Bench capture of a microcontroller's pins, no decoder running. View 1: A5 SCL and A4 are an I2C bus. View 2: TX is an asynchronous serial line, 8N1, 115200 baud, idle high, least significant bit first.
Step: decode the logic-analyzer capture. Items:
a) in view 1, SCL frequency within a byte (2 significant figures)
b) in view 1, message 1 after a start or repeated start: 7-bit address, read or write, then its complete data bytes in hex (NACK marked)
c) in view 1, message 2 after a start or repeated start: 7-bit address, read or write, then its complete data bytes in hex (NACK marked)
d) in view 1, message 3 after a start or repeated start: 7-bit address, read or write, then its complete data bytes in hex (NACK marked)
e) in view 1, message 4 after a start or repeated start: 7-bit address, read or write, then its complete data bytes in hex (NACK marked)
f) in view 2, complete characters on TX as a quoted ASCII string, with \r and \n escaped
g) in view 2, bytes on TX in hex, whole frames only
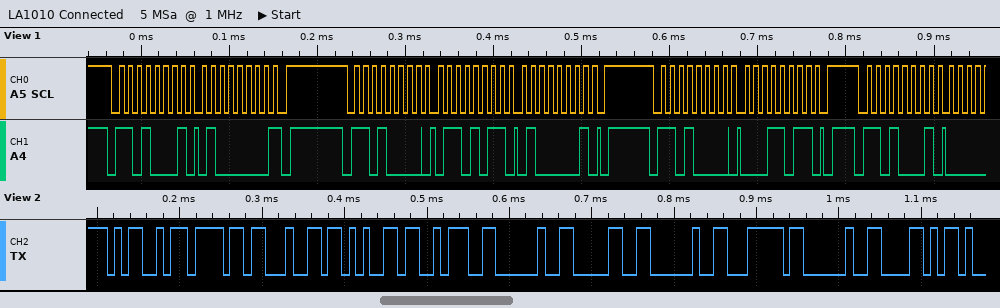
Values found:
100 kHz
0x68 read: 40 NACK
0x68 write: 6B 41
0x68 write: 1B
0x68 read
"Mode: 0 | X"
4D 6F 64 65 3A 20 30 20 7C 20 58
